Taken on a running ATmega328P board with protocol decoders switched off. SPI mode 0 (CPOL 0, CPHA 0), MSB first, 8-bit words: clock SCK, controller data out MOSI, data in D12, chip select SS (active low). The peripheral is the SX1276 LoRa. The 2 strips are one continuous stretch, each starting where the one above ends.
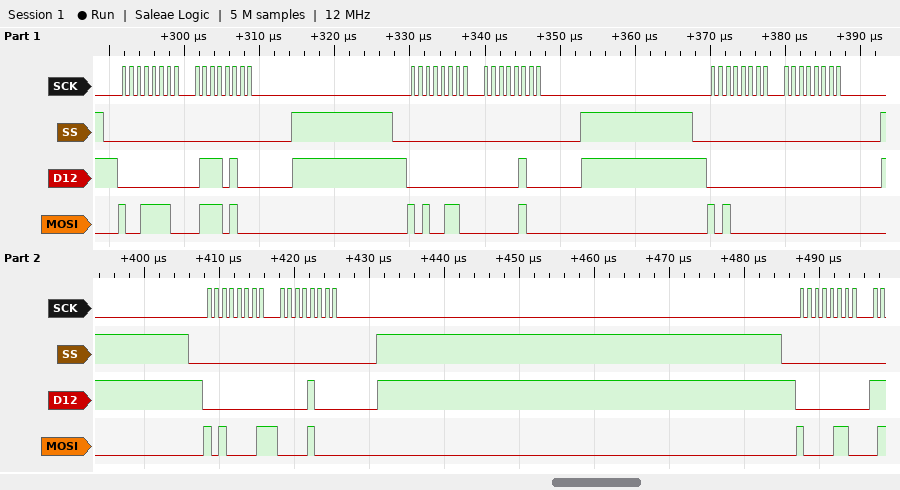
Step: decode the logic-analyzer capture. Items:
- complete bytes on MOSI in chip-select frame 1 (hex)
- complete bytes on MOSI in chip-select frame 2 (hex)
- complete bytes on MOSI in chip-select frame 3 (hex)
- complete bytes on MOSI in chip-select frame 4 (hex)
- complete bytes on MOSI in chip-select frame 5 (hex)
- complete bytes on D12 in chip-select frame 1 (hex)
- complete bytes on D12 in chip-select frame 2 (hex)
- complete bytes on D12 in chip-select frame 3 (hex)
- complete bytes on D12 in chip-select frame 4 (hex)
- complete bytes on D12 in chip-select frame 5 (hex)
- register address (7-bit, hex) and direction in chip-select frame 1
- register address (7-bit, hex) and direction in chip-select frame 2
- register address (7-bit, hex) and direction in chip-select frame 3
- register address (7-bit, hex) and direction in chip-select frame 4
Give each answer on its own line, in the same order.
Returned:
9E 74
A6 04
A0 00
A1 08
86
00 74
00 04
00 00
00 08
00
0x1E write
0x26 write
0x20 write
0x21 write
